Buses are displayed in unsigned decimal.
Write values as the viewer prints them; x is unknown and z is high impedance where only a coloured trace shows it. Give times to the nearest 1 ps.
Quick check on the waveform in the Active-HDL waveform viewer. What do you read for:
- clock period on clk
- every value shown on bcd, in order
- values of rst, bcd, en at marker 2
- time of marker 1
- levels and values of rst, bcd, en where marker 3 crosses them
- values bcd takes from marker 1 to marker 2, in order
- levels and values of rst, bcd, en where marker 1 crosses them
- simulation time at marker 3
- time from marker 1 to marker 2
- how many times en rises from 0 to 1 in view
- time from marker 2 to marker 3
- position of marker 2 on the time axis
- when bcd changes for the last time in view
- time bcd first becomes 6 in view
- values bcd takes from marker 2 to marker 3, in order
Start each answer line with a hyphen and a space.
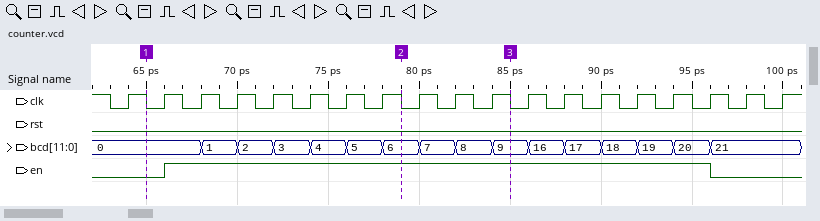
- 2 ps
- 0, 1, 2, 3, 4, 5, 6, 7, 8, 9, 16, 17, 18, 19, 20, 21
- rst=0, bcd=6, en=1
- 65 ps
- rst=0, bcd=9, en=1
- 0, 1, 2, 3, 4, 5, 6
- rst=0, bcd=0, en=0
- 85 ps
- 14 ps
- 1
- 6 ps
- 79 ps
- 96 ps
- 78 ps
- 6, 7, 8, 9
